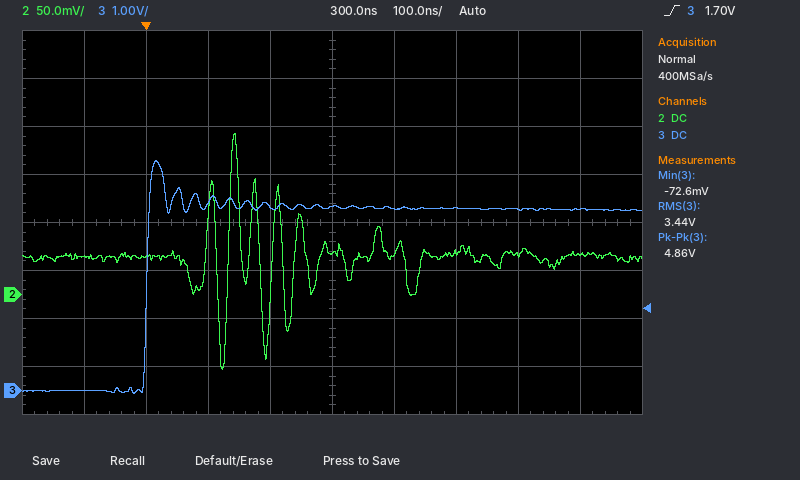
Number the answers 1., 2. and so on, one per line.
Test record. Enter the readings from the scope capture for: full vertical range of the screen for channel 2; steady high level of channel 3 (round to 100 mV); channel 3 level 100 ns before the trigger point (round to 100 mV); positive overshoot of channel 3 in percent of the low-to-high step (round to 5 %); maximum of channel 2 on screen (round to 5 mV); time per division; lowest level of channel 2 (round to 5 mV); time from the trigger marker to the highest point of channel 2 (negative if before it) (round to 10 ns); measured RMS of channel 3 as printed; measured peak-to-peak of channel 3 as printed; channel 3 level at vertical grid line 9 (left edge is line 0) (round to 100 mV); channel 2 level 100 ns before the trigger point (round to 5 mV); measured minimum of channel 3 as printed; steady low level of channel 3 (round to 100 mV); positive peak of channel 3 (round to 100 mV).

1. 400 mV
2. 3.8 V
3. 0.0 V
4. 25 %
5. 170 mV
6. 100 ns
7. -80 mV
8. +140 ns
9. 3.44 V
10. 4.86 V
11. 3.8 V
12. 40 mV
13. -72.6 mV
14. 0.0 V
15. 4.8 V
